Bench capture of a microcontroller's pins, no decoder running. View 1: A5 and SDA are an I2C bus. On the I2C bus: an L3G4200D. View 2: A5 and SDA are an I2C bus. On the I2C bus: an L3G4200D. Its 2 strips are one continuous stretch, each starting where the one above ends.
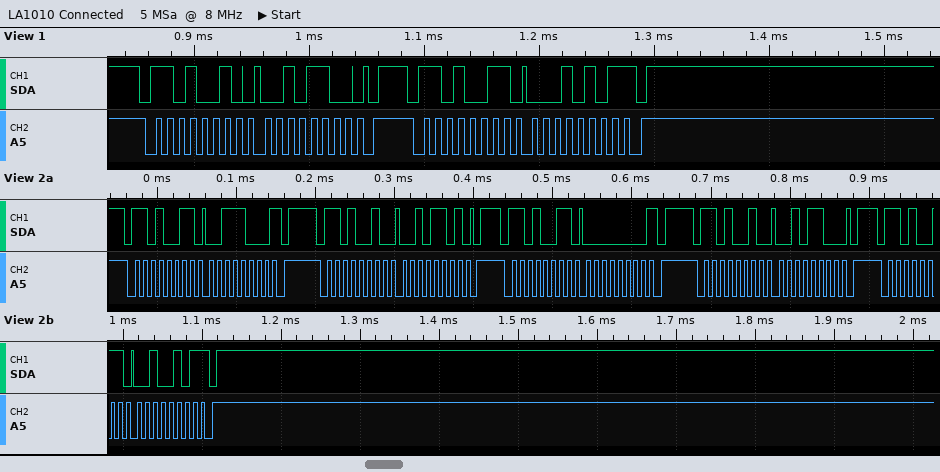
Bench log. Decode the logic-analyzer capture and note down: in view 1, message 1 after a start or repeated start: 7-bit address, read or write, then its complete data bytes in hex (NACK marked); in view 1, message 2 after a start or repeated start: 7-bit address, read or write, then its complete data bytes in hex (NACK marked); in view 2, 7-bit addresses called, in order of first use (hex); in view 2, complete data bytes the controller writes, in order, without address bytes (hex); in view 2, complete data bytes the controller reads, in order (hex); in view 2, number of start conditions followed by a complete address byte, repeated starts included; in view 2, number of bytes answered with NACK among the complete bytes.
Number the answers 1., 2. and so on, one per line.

1. 0x69 write: 2C
2. 0x69 read: 15 NACK
3. 0x69
4. 2D 2C
5. 38 00 25
6. 5
7. 3
